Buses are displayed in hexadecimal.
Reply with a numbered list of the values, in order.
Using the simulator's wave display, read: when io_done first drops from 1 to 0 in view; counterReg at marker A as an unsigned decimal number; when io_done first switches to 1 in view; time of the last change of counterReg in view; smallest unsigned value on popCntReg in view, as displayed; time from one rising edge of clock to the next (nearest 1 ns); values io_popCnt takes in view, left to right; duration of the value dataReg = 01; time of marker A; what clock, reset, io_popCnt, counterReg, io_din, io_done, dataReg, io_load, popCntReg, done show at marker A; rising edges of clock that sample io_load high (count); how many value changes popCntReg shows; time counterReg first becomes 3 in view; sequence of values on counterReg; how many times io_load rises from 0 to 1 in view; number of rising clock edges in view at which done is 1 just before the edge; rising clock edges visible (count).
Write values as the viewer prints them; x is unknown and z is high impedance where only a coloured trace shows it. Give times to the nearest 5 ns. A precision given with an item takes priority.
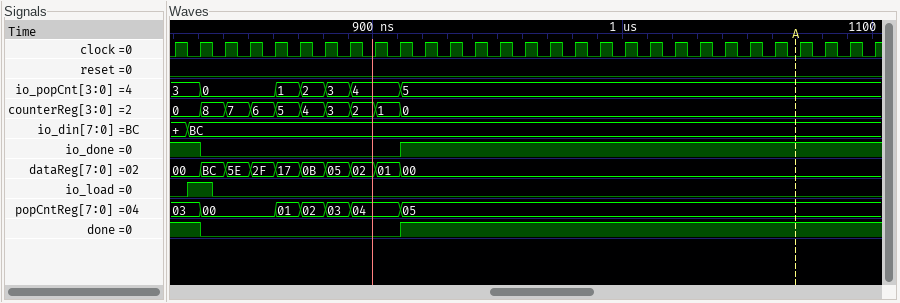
1. 830 ns
2. 0
3. 910 ns
4. 910 ns
5. 00
6. 10 ns
7. 3, 0, 1, 2, 3, 4, 5
8. 10 ns
9. 1070 ns
10. clock=0, reset=0, io_popCnt=5, counterReg=0, io_din=BC, io_done=1, dataReg=00, io_load=0, popCntReg=05, done=1
11. 1
12. 6
13. 880 ns
14. 0, 8, 7, 6, 5, 4, 3, 2, 1, 0
15. 1
16. 21
17. 29
